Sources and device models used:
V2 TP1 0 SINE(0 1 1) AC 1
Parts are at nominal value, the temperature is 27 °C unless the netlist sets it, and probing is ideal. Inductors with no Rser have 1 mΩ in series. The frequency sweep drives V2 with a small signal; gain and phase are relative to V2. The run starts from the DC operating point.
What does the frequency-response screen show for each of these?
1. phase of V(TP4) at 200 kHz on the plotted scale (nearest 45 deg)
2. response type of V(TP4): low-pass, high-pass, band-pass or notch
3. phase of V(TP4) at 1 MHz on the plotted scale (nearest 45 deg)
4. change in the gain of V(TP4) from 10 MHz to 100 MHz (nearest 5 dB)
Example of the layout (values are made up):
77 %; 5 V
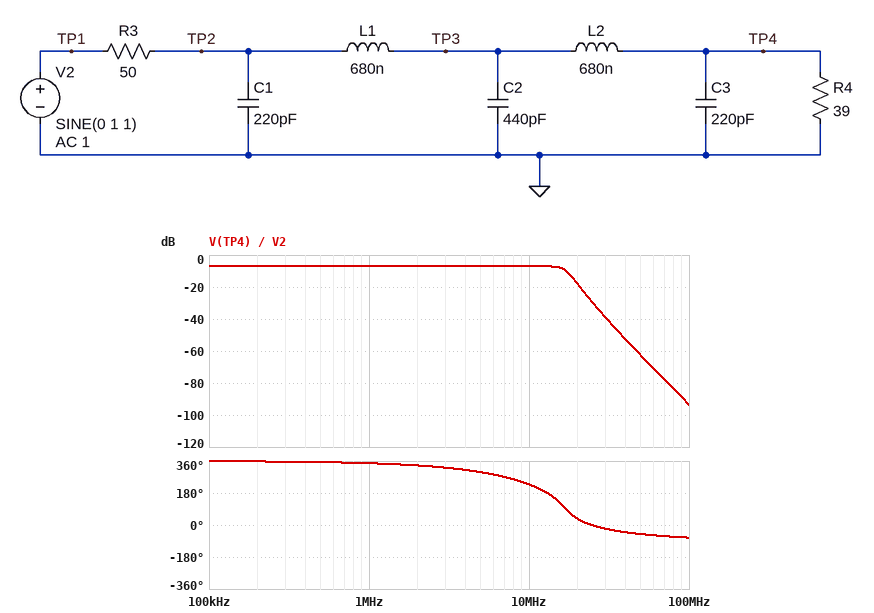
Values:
360 deg; low-pass; 360 deg; -85 dB
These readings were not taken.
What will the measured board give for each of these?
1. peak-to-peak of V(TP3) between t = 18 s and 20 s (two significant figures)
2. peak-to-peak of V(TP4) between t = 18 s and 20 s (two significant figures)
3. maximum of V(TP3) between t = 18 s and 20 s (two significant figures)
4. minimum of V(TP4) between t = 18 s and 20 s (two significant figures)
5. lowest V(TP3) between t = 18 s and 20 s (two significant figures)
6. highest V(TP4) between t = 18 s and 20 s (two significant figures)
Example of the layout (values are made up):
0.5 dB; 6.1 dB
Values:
880 mV; 880 mV; 440 mV; -440 mV; -440 mV; 440 mV
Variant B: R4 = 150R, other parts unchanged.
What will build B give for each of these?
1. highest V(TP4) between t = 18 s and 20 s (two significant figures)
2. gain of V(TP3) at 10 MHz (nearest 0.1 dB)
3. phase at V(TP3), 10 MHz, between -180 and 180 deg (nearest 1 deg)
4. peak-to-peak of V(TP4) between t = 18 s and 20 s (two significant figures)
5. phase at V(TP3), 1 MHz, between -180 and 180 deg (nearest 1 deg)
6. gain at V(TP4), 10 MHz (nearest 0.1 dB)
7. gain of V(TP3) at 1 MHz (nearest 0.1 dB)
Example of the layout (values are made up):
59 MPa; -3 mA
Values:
750 mV; -8.7 dB; -96 deg; 1.5 V; -13 deg; -2.7 dB; -2.6 dB
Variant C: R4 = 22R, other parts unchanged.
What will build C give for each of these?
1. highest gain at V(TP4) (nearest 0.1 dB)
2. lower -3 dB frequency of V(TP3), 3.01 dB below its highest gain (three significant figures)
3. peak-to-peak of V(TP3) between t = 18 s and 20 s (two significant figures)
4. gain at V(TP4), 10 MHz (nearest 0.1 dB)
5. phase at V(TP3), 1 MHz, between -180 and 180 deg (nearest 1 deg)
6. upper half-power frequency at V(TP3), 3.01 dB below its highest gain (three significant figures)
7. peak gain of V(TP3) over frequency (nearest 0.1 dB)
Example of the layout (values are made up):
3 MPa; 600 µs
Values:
-9.8 dB; 9.53 MHz; 610 mV; -10.2 dB; -1 deg; 17.4 MHz; -1.5 dB
